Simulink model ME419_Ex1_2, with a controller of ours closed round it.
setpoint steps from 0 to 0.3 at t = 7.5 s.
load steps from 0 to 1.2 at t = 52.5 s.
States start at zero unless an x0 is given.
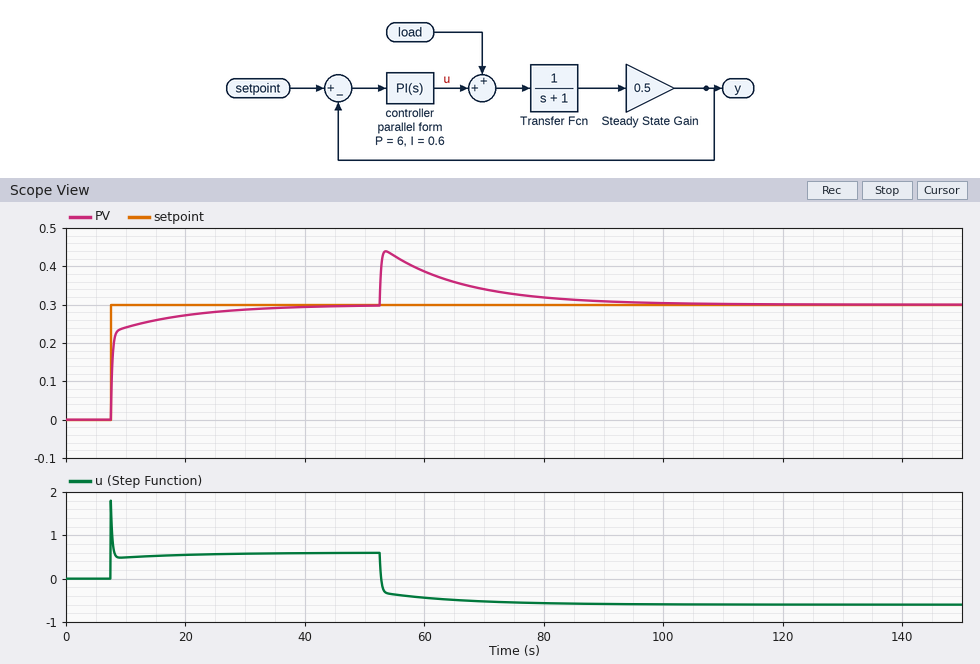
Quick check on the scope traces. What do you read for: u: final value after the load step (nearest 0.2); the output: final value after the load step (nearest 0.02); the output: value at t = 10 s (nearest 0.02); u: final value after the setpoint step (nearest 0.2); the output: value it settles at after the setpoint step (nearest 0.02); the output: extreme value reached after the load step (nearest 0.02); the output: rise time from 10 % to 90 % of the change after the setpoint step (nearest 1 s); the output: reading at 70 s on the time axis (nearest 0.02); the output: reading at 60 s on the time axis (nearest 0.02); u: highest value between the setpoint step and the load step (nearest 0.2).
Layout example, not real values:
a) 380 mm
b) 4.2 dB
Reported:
a) -0.6
b) 0.30
c) 0.24
d) 0.6
e) 0.30
f) 0.44
g) 11 s
h) 0.34
i) 0.38
j) 1.8
